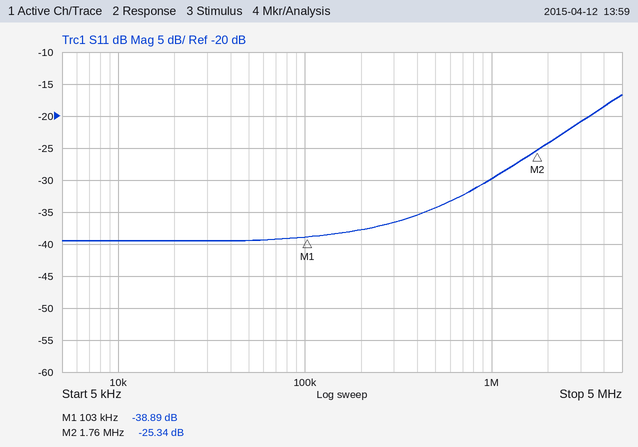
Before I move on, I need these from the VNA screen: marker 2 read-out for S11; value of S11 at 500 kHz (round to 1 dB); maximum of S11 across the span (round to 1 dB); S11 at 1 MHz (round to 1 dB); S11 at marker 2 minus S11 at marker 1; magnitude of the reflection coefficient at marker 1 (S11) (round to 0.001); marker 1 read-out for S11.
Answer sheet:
-25.34 dB
-34 dB
-17 dB
-30 dB
13.55 dB
0.011
-38.89 dB
